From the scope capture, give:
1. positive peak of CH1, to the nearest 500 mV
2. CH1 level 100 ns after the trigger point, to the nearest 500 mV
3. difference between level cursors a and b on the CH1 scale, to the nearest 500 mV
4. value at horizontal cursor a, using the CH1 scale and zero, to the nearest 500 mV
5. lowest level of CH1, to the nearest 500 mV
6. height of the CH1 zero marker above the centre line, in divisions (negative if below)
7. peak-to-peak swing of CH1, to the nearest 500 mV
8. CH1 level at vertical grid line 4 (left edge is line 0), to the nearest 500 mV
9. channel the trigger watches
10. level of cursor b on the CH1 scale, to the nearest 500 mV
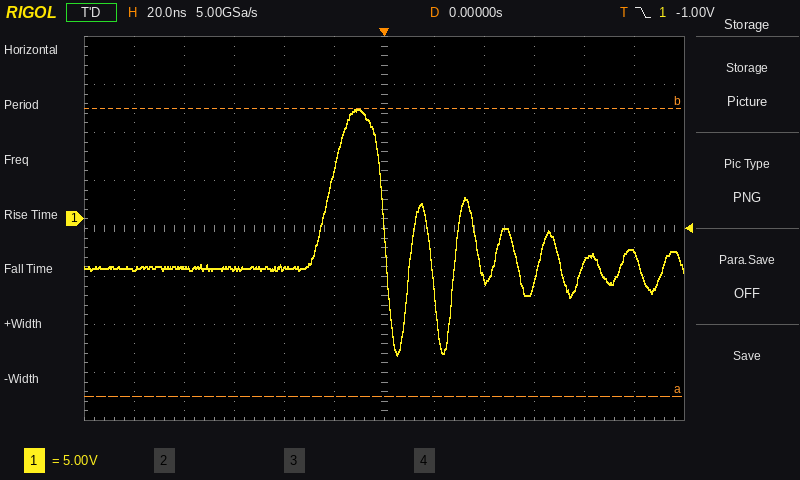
11.5 V
-3.5 V
30.0 V
-18.5 V
-14.0 V
+0.2 div
25.5 V
-5.0 V
CH1
11.5 V
